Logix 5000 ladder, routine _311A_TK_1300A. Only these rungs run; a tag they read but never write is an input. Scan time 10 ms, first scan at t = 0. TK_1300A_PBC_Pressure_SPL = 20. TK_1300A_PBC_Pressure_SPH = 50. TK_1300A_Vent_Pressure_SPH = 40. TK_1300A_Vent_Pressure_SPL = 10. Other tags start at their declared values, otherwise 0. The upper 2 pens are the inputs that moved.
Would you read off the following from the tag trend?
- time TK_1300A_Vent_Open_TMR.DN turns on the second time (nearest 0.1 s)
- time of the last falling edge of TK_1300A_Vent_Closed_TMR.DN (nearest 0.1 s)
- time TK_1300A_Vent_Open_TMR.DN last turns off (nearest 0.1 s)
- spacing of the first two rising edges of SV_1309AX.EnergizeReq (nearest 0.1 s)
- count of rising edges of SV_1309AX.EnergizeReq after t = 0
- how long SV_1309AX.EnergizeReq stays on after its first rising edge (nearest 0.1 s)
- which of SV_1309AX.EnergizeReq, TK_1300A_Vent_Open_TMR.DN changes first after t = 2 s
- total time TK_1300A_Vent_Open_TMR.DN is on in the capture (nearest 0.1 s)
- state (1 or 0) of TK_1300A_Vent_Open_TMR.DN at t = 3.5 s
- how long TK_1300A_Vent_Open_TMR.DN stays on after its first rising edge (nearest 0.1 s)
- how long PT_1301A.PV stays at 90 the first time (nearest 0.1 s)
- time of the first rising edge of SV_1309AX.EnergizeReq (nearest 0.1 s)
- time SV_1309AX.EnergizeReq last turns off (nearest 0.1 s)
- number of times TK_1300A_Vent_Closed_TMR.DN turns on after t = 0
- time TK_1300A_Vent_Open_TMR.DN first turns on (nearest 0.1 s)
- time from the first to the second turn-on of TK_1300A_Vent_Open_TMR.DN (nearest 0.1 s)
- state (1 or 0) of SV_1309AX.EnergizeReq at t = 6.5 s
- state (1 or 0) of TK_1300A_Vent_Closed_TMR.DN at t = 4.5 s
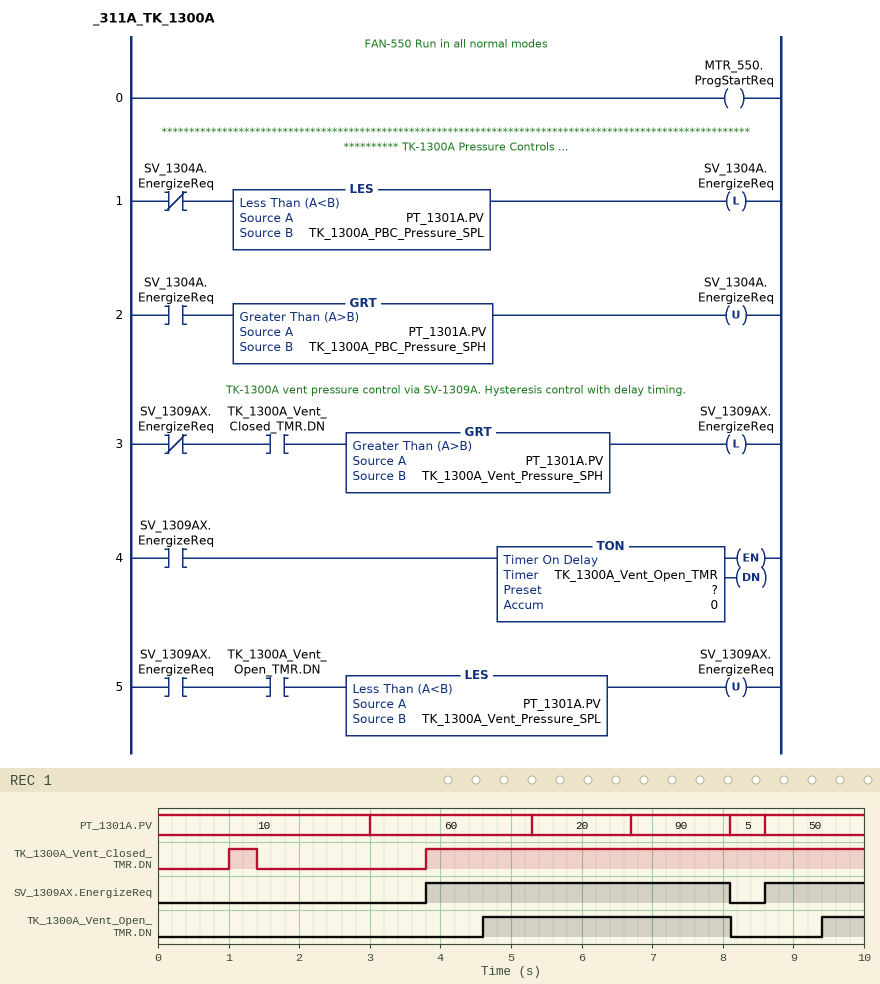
9.4 s
1.4 s
8.1 s
4.8 s
2
4.3 s
SV_1309AX.EnergizeReq
4.1 s
0
3.5 s
1.4 s
3.8 s
8.1 s
2
4.6 s
4.8 s
1
1
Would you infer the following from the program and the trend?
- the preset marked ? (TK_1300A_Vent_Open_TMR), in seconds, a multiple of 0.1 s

0.8 s
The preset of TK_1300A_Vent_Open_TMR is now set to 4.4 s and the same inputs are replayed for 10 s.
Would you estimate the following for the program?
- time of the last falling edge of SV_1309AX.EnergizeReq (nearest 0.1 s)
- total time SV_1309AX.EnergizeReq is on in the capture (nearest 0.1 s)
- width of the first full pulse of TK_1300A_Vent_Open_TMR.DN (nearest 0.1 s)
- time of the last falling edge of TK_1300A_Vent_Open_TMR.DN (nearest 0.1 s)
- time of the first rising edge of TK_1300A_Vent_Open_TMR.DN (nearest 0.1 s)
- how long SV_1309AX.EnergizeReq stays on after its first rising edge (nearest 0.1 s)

8.2 s
5.8 s
0.0 s
8.2 s
8.2 s
4.4 s
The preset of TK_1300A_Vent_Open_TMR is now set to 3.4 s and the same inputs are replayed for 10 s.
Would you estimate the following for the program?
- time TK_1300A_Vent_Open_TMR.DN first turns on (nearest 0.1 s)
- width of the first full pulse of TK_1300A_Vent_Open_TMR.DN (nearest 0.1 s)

7.2 s
0.9 s
